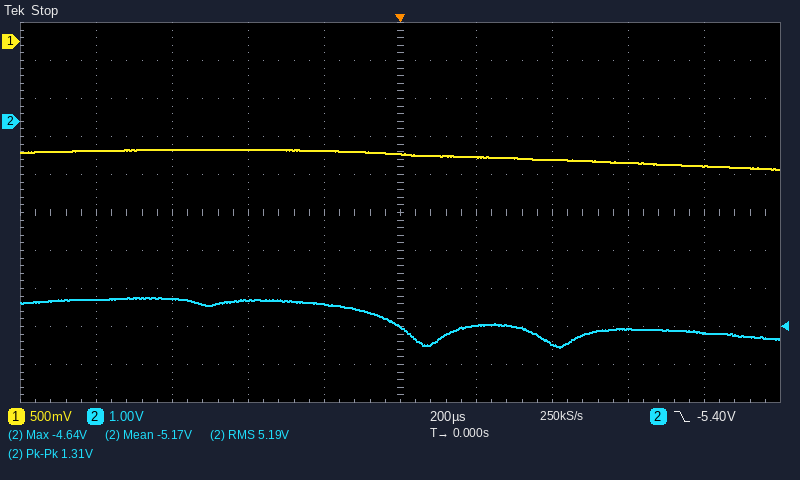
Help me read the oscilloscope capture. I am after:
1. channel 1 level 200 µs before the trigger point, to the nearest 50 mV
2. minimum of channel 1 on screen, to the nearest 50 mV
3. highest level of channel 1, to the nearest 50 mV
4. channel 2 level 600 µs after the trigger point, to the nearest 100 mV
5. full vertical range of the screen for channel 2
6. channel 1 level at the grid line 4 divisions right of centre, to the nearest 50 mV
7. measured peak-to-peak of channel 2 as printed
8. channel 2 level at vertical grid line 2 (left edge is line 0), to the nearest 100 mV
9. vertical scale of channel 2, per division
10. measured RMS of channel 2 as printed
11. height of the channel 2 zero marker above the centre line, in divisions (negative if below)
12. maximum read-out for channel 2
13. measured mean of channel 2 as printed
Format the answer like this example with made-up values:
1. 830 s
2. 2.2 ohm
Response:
1. -1.45 V
2. -1.70 V
3. -1.40 V
4. -5.5 V
5. 10 V
6. -1.65 V
7. 1.31 V
8. -4.7 V
9. 1 V
10. 5.19 V
11. +2.4 div
12. -4.64 V
13. -5.17 V
